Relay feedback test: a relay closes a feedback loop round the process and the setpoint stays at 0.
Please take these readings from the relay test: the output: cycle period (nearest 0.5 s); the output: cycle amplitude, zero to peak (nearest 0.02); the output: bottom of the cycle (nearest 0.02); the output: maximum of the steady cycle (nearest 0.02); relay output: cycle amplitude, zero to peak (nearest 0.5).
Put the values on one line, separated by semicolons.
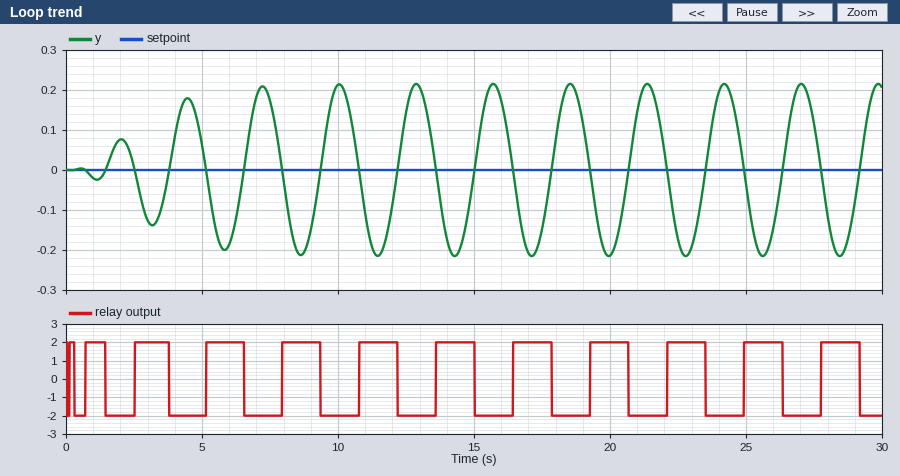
3.0 s; 0.22; -0.22; 0.22; 2.0
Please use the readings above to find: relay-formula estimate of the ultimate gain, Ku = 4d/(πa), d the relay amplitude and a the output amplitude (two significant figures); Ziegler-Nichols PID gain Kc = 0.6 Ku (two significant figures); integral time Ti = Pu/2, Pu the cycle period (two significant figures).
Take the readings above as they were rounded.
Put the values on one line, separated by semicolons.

12; 7.2; 1.5 s
